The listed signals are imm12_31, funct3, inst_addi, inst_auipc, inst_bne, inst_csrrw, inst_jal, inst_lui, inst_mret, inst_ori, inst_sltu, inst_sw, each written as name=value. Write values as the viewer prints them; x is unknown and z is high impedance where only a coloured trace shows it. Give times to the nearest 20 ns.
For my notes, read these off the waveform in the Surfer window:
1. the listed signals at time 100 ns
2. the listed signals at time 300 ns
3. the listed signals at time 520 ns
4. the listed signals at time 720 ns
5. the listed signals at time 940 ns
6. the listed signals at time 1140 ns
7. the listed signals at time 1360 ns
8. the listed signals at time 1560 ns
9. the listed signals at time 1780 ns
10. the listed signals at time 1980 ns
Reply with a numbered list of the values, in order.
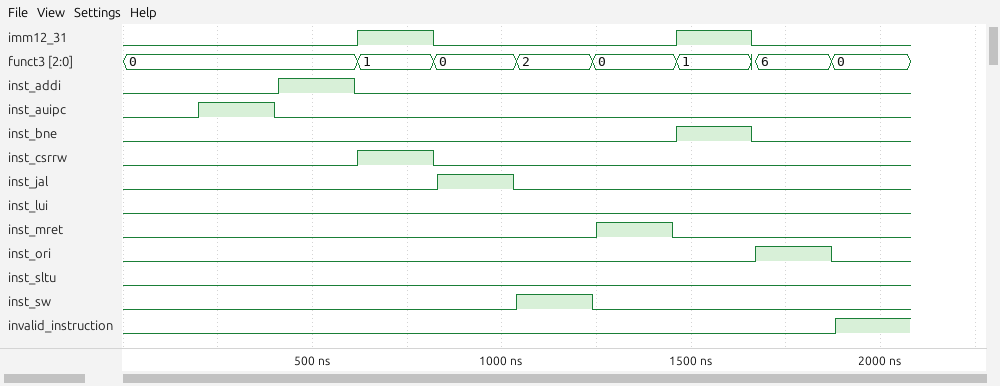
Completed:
1. imm12_31=0, funct3=0, inst_addi=0, inst_auipc=0, inst_bne=0, inst_csrrw=0, inst_jal=0, inst_lui=0, inst_mret=0, inst_ori=0, inst_sltu=0, inst_sw=0
2. imm12_31=0, funct3=0, inst_addi=0, inst_auipc=1, inst_bne=0, inst_csrrw=0, inst_jal=0, inst_lui=0, inst_mret=0, inst_ori=0, inst_sltu=0, inst_sw=0
3. imm12_31=0, funct3=0, inst_addi=1, inst_auipc=0, inst_bne=0, inst_csrrw=0, inst_jal=0, inst_lui=0, inst_mret=0, inst_ori=0, inst_sltu=0, inst_sw=0
4. imm12_31=1, funct3=1, inst_addi=0, inst_auipc=0, inst_bne=0, inst_csrrw=1, inst_jal=0, inst_lui=0, inst_mret=0, inst_ori=0, inst_sltu=0, inst_sw=0
5. imm12_31=0, funct3=0, inst_addi=0, inst_auipc=0, inst_bne=0, inst_csrrw=0, inst_jal=1, inst_lui=0, inst_mret=0, inst_ori=0, inst_sltu=0, inst_sw=0
6. imm12_31=0, funct3=2, inst_addi=0, inst_auipc=0, inst_bne=0, inst_csrrw=0, inst_jal=0, inst_lui=0, inst_mret=0, inst_ori=0, inst_sltu=0, inst_sw=1
7. imm12_31=0, funct3=0, inst_addi=0, inst_auipc=0, inst_bne=0, inst_csrrw=0, inst_jal=0, inst_lui=0, inst_mret=1, inst_ori=0, inst_sltu=0, inst_sw=0
8. imm12_31=1, funct3=1, inst_addi=0, inst_auipc=0, inst_bne=1, inst_csrrw=0, inst_jal=0, inst_lui=0, inst_mret=0, inst_ori=0, inst_sltu=0, inst_sw=0
9. imm12_31=0, funct3=6, inst_addi=0, inst_auipc=0, inst_bne=0, inst_csrrw=0, inst_jal=0, inst_lui=0, inst_mret=0, inst_ori=1, inst_sltu=0, inst_sw=0
10. imm12_31=0, funct3=0, inst_addi=0, inst_auipc=0, inst_bne=0, inst_csrrw=0, inst_jal=0, inst_lui=0, inst_mret=0, inst_ori=0, inst_sltu=0, inst_sw=0
